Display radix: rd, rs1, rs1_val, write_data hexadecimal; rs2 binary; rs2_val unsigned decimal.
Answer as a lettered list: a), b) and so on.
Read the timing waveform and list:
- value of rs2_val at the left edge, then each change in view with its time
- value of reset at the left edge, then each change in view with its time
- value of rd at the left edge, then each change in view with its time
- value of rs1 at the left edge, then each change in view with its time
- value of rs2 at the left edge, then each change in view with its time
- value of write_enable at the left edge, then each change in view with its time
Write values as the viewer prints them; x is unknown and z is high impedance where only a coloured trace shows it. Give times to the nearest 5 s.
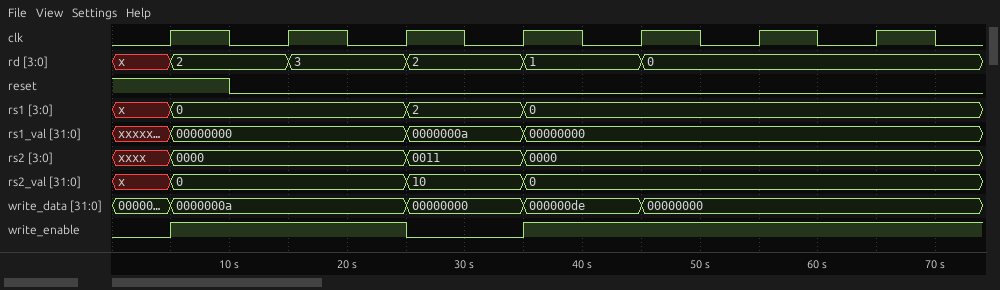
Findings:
a) x, 0 at 5 s, 10 at 25 s, 0 at 35 s
b) 1, 0 at 10 s
c) x, 2 at 5 s, 3 at 15 s, 2 at 25 s, 1 at 35 s, 0 at 45 s
d) x, 0 at 5 s, 2 at 25 s, 0 at 35 s
e) xxxx, 0000 at 5 s, 0011 at 25 s, 0000 at 35 s
f) 0, 1 at 5 s, 0 at 25 s, 1 at 35 s
